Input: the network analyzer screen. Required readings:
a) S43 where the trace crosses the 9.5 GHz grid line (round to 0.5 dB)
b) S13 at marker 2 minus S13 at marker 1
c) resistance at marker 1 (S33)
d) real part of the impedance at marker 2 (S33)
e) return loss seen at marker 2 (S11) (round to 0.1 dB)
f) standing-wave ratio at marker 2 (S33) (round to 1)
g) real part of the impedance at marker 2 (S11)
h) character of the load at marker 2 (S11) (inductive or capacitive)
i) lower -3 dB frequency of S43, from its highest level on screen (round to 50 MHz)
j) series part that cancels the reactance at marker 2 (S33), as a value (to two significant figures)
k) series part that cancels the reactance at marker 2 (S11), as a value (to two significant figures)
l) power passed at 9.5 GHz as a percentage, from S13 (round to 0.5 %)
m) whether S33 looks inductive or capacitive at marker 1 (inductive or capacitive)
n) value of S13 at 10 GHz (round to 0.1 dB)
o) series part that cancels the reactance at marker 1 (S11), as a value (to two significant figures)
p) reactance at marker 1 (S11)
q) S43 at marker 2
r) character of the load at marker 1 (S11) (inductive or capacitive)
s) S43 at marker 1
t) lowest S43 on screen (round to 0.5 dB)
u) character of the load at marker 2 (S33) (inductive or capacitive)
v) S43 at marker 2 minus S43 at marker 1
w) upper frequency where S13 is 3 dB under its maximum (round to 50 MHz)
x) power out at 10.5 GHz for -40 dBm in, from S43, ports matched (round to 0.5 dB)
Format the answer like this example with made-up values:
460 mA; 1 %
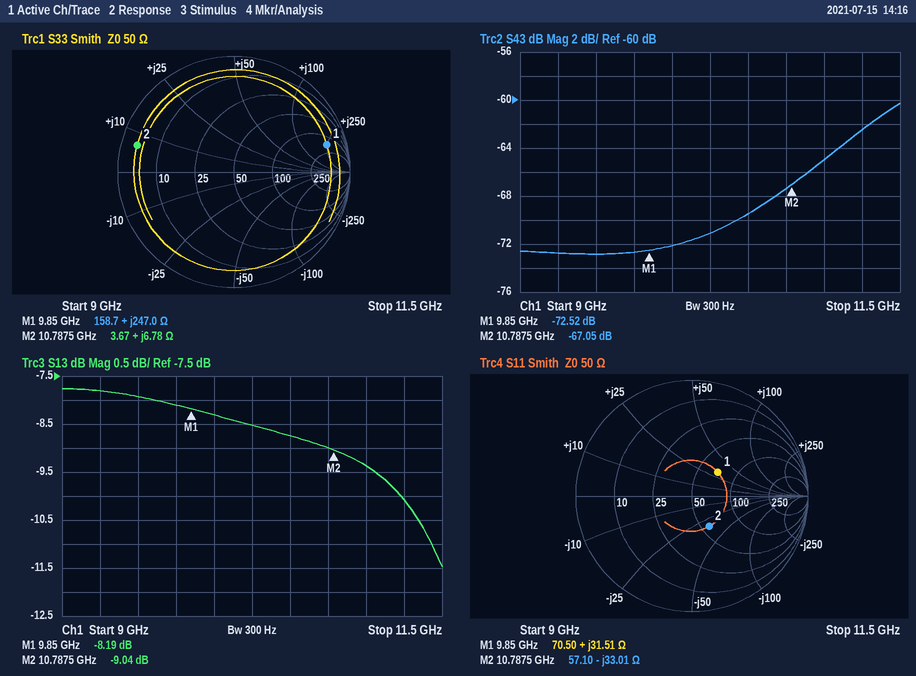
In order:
-73.0 dB; -0.85 dB; 158.7 Ω; 3.67 Ω; 10.4 dB; 14; 57.10 Ω; capacitive; 11.15 GHz; 2.2 pF; 490 pH; 16.0 %; inductive; -8.3 dB; 510 fF; +31.51 Ω; -67.05 dB; inductive; -72.52 dB; -73.0 dB; inductive; 5.47 dB; 11.40 GHz; -109.5 dBm
